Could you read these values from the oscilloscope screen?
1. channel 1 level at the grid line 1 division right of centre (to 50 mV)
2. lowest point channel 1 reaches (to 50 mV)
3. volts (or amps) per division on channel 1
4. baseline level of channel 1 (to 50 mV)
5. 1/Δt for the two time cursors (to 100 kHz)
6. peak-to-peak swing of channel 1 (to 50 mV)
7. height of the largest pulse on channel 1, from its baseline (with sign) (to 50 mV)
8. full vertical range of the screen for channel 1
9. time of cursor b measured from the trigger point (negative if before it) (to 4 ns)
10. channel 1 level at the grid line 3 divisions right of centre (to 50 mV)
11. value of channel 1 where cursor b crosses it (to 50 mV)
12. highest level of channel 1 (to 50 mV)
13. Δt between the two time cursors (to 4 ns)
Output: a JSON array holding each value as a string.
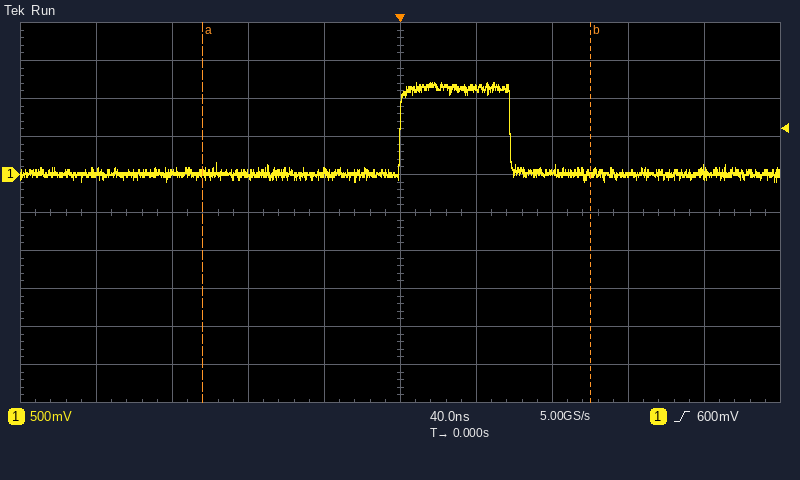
["1.15 V", "-100 mV", "500 mV", "0 mV", "4.9 MHz", "1.30 V", "+1.20 V", "5 V", "+100 ns", "0 mV", "0 mV", "1.20 V", "204 ns"]
